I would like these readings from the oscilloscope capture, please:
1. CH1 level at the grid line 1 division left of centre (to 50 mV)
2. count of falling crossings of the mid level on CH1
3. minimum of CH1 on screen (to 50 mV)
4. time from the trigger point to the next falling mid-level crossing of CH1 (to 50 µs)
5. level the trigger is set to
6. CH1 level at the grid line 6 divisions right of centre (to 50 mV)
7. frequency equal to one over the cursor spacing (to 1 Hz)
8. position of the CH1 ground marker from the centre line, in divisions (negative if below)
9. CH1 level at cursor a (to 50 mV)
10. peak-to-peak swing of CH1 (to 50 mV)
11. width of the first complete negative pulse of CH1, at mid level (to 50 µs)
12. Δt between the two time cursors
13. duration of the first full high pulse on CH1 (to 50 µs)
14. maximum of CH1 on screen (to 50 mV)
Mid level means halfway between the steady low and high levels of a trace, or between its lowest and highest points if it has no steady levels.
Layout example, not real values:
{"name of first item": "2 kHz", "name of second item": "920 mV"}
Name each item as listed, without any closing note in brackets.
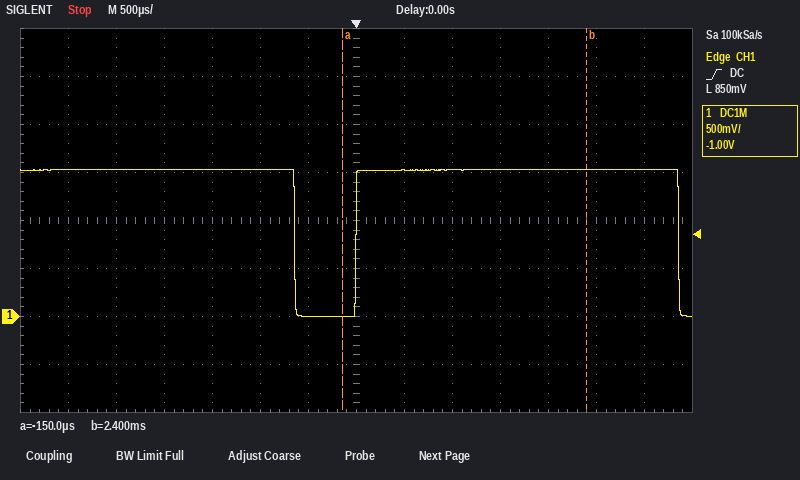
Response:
{"CH1 level at the grid line 1 division left of centre": "0 mV", "count of falling crossings of the mid level on CH1": "2", "minimum of CH1 on screen": "0 mV", "time from the trigger point to the next falling mid-level crossing of CH1": "3.35 ms", "level the trigger is set to": "850 mV", "CH1 level at the grid line 6 divisions right of centre": "1.55 V", "frequency equal to one over the cursor spacing": "392 Hz", "position of the CH1 ground marker from the centre line, in divisions": "-2.0 div", "CH1 level at cursor a": "0 mV", "peak-to-peak swing of CH1": "1.55 V", "width of the first complete negative pulse of CH1, at mid level": "650 µs", "Δt between the two time cursors": "2.55 ms", "duration of the first full high pulse on CH1": "3.35 ms", "maximum of CH1 on screen": "1.55 V"}
